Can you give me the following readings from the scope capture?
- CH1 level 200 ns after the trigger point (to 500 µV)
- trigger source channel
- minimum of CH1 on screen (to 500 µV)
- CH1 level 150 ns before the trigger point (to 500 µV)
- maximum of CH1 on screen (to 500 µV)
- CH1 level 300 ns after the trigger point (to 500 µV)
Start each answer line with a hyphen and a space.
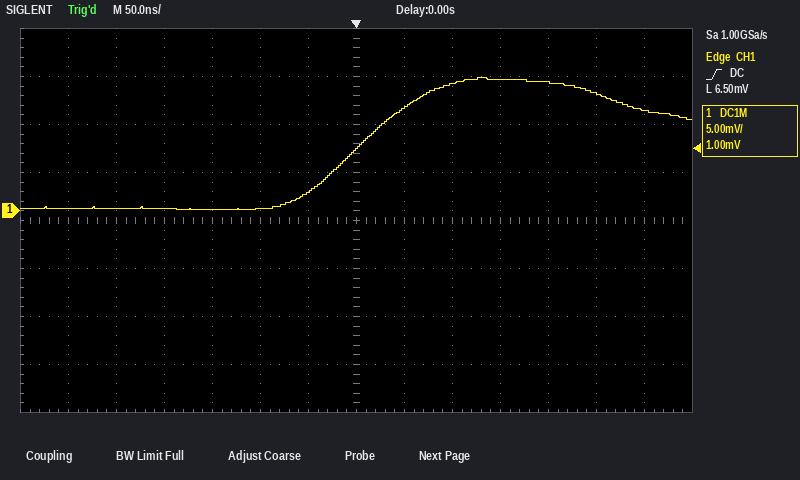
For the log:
- 13.5 mV
- CH1
- 0.0 mV
- 0.0 mV
- 14.0 mV
- 10.5 mV
